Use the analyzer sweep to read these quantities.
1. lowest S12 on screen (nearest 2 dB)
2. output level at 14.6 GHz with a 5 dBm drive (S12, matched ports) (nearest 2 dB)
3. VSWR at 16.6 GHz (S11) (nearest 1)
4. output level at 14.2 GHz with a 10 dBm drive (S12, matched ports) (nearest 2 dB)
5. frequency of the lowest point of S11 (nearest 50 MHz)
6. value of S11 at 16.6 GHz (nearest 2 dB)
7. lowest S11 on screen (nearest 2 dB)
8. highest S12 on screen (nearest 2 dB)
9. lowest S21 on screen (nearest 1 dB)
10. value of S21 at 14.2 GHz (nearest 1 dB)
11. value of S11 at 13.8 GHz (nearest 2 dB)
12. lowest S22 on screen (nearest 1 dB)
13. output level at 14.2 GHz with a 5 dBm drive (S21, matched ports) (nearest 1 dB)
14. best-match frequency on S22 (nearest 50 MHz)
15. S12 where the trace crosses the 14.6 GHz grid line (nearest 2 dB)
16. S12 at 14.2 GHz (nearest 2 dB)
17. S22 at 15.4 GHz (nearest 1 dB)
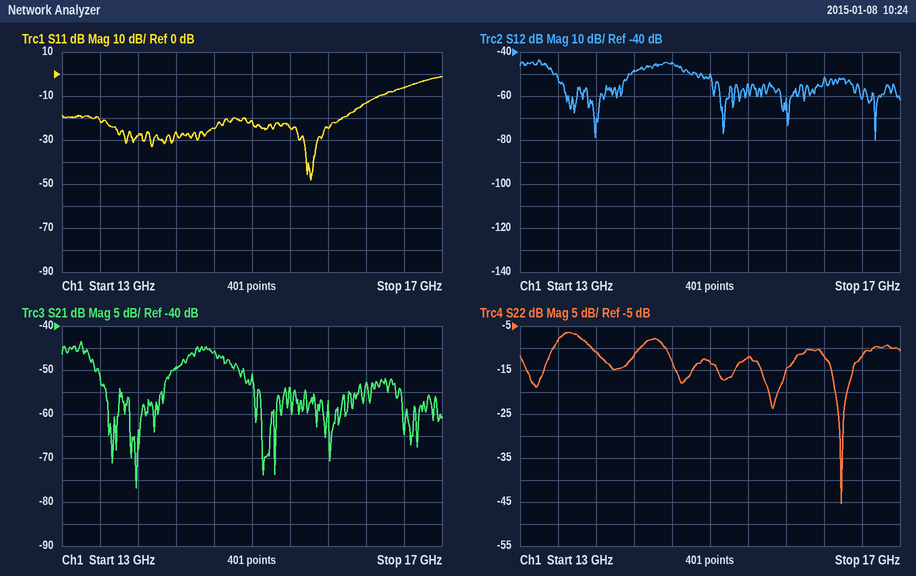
-80 dB
-40 dBm
3
-38 dBm
15.60 GHz
-6 dB
-48 dB
-44 dB
-77 dB
-49 dB
-28 dB
-45 dB
-44 dBm
16.40 GHz
-44 dB
-48 dB
-12 dB
